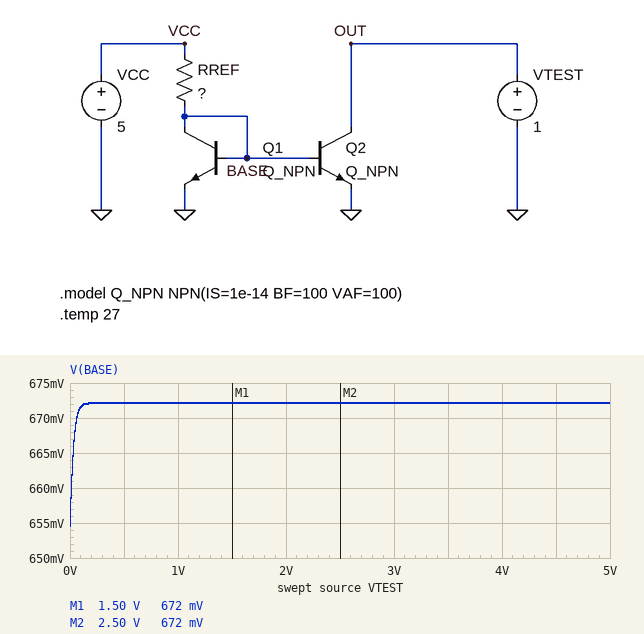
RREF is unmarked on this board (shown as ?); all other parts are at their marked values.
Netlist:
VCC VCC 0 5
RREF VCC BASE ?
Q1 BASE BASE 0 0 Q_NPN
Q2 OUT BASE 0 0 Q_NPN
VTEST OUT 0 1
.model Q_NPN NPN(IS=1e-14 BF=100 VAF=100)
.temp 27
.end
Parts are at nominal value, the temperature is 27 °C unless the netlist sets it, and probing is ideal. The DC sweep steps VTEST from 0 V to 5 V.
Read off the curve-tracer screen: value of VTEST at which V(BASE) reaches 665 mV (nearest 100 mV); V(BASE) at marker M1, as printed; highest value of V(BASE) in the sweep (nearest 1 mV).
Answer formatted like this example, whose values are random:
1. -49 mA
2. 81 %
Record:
1. 0 V
2. 672 mV
3. 672 mV
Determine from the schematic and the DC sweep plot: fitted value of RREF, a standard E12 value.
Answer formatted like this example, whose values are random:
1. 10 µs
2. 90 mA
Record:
1. 2.2 kΩ
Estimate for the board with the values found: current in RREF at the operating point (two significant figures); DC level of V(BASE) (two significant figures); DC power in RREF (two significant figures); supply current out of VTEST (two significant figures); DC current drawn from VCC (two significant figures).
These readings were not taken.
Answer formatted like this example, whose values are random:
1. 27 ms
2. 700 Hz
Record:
1. 2.0 mA
2. 670 mV
3. 8.5 mW
4. 1.9 mA
5. 2.0 mA
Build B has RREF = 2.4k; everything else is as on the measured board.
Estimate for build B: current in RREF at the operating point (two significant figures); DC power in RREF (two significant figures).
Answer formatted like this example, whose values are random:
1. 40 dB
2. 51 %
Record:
1. 1.8 mA
2. 7.8 mW
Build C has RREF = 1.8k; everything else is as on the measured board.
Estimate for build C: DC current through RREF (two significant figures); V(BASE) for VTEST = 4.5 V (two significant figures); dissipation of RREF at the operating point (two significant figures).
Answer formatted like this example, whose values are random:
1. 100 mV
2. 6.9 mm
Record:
1. 2.4 mA
2. 680 mV
3. 10 mW
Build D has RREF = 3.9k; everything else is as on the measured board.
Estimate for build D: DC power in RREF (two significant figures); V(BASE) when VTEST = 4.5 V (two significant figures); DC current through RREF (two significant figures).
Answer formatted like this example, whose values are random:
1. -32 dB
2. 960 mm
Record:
1. 4.8 mW
2. 660 mV
3. 1.1 mA
